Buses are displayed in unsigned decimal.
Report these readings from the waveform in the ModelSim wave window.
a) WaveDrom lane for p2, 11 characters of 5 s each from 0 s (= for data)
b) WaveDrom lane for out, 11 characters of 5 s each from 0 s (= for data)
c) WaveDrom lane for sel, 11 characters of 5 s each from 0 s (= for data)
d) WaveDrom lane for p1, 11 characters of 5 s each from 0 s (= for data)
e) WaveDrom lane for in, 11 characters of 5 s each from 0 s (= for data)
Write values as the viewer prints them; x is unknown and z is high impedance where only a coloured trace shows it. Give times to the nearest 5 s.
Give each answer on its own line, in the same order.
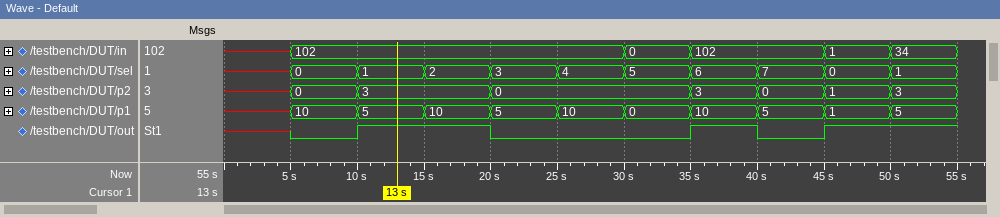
{name: 'p2', wave: 'x==.=..====', data: '0 3 0 3 0 1 3'}
{name: 'out', wave: 'x01.0..101.'}
{name: 'sel', wave: 'x==========', data: '0 1 2 3 4 5 6 7 0 1'}
{name: 'p1', wave: 'x==========', data: '10 5 10 5 10 0 10 5 1 5'}
{name: 'in', wave: 'x=....==.==', data: '102 0 102 1 34'}
